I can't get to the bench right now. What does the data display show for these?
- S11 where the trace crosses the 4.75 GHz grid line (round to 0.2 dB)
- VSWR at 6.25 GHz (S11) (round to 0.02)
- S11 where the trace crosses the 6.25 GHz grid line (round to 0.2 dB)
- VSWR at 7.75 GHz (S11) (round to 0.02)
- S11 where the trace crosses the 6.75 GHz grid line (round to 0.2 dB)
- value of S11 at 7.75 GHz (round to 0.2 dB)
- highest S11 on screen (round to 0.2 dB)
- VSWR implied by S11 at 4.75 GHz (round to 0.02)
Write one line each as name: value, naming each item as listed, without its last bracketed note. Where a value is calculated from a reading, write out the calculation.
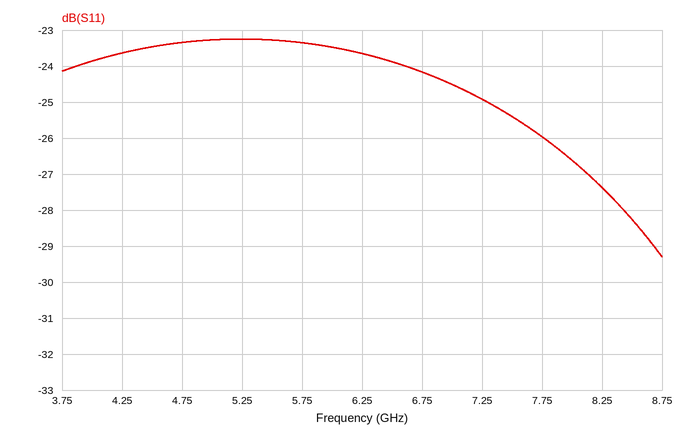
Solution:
S11 where the trace crosses the 4.75 GHz grid line: -23.4 dB
VSWR at 6.25 GHz (S11): |Γ| = 10^(-23.6/20) = 0.0661; VSWR = (1 + 0.0661)/(1 − 0.0661) ≈ 1.14
S11 where the trace crosses the 6.25 GHz grid line: -23.6 dB
VSWR at 7.75 GHz (S11): |Γ| = 10^(-26/20) = 0.0501; VSWR = (1 + 0.0501)/(1 − 0.0501) ≈ 1.11, so 1.10 to the nearest 0.02
S11 where the trace crosses the 6.75 GHz grid line: -24.2 dB
value of S11 at 7.75 GHz: -26.0 dB
highest S11 on screen: -23.2 dB
VSWR implied by S11 at 4.75 GHz: |Γ| = 10^(-23.4/20) = 0.0676; VSWR = (1 + 0.0676)/(1 − 0.0676) ≈ 1.15, so 1.14 to the nearest 0.02
